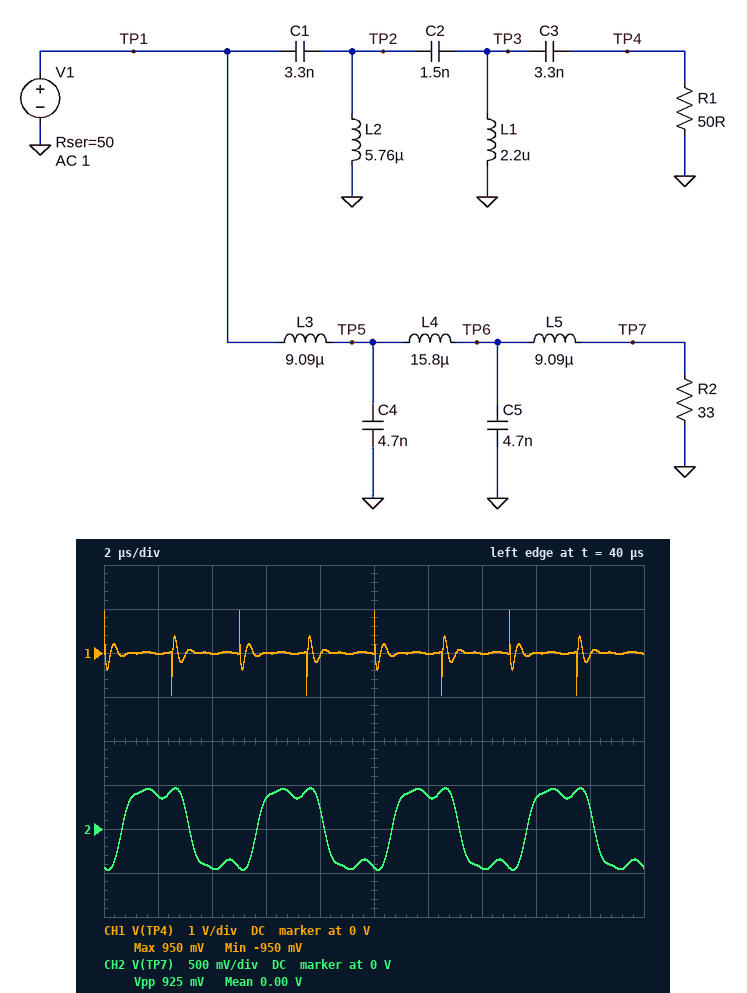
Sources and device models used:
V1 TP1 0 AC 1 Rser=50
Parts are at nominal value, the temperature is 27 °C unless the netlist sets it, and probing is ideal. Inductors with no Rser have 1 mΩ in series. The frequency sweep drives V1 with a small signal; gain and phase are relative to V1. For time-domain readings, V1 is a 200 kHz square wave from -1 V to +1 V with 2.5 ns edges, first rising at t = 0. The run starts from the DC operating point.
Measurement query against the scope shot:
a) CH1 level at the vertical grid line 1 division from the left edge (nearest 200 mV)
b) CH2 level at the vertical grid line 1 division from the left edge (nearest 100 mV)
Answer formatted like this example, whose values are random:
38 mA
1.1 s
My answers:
0 V
400 mV
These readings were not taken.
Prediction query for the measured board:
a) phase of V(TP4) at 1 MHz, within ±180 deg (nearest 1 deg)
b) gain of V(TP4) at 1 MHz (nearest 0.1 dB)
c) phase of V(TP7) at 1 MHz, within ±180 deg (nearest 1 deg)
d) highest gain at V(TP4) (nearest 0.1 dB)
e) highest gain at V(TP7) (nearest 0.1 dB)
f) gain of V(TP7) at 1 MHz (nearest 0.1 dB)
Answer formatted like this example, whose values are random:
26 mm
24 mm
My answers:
-87 deg
-18.1 dB
166 deg
-6.0 dB
-8.0 dB
-14.2 dB
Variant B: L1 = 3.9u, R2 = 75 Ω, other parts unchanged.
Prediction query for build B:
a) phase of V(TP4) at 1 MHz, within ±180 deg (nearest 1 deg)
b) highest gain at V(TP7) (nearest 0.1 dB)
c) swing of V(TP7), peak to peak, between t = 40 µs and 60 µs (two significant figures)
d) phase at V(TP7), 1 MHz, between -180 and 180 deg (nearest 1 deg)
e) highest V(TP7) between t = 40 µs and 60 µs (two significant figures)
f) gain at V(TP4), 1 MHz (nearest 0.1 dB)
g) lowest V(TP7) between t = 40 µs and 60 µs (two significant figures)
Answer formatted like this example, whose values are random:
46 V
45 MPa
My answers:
-132 deg
-4.4 dB
1.4 V
145 deg
700 mV
-12.8 dB
-700 mV
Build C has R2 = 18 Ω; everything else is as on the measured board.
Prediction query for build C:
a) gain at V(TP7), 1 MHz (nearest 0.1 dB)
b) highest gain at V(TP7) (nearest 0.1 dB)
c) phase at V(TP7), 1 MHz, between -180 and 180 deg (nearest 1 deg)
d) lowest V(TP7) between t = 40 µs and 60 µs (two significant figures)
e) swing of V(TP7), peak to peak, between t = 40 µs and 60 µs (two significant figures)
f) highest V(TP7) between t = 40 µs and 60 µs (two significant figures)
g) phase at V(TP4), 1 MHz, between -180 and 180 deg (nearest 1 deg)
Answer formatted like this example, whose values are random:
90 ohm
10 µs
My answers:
-19.1 dB
-11.4 dB
165 deg
-310 mV
620 mV
310 mV
-79 deg
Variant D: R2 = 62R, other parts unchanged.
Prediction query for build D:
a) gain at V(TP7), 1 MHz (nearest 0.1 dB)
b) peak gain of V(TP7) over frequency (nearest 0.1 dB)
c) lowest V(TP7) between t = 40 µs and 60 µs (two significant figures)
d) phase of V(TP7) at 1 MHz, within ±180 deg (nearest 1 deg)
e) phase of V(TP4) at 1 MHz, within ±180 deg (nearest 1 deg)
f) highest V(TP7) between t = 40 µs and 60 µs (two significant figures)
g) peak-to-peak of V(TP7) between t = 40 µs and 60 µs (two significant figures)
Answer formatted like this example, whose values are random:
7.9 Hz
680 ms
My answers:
-9.4 dB
-5.1 dB
-660 mV
168 deg
-100 deg
660 mV
1.3 V
